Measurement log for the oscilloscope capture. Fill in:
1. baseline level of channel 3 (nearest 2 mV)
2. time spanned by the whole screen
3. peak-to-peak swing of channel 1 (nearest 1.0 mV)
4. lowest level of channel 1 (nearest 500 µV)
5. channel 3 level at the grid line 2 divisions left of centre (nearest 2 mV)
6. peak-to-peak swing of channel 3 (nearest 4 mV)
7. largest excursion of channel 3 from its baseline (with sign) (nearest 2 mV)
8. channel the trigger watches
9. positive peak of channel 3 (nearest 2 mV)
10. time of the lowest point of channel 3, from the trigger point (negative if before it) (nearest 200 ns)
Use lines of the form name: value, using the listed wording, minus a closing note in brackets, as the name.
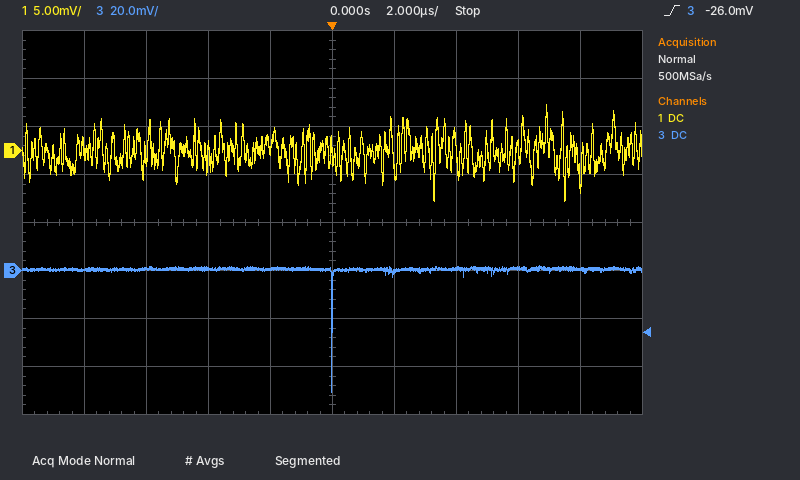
baseline level of channel 3: 0 mV
time spanned by the whole screen: 20 µs
peak-to-peak swing of channel 1: 10.0 mV
lowest level of channel 1: -5.5 mV
channel 3 level at the grid line 2 divisions left of centre: 0 mV
peak-to-peak swing of channel 3: 52 mV
largest excursion of channel 3 from its baseline (with sign): -52 mV
channel the trigger watches: channel 3
positive peak of channel 3: 2 mV
time of the lowest point of channel 3, from the trigger point (negative if before it): 0.0 µs
